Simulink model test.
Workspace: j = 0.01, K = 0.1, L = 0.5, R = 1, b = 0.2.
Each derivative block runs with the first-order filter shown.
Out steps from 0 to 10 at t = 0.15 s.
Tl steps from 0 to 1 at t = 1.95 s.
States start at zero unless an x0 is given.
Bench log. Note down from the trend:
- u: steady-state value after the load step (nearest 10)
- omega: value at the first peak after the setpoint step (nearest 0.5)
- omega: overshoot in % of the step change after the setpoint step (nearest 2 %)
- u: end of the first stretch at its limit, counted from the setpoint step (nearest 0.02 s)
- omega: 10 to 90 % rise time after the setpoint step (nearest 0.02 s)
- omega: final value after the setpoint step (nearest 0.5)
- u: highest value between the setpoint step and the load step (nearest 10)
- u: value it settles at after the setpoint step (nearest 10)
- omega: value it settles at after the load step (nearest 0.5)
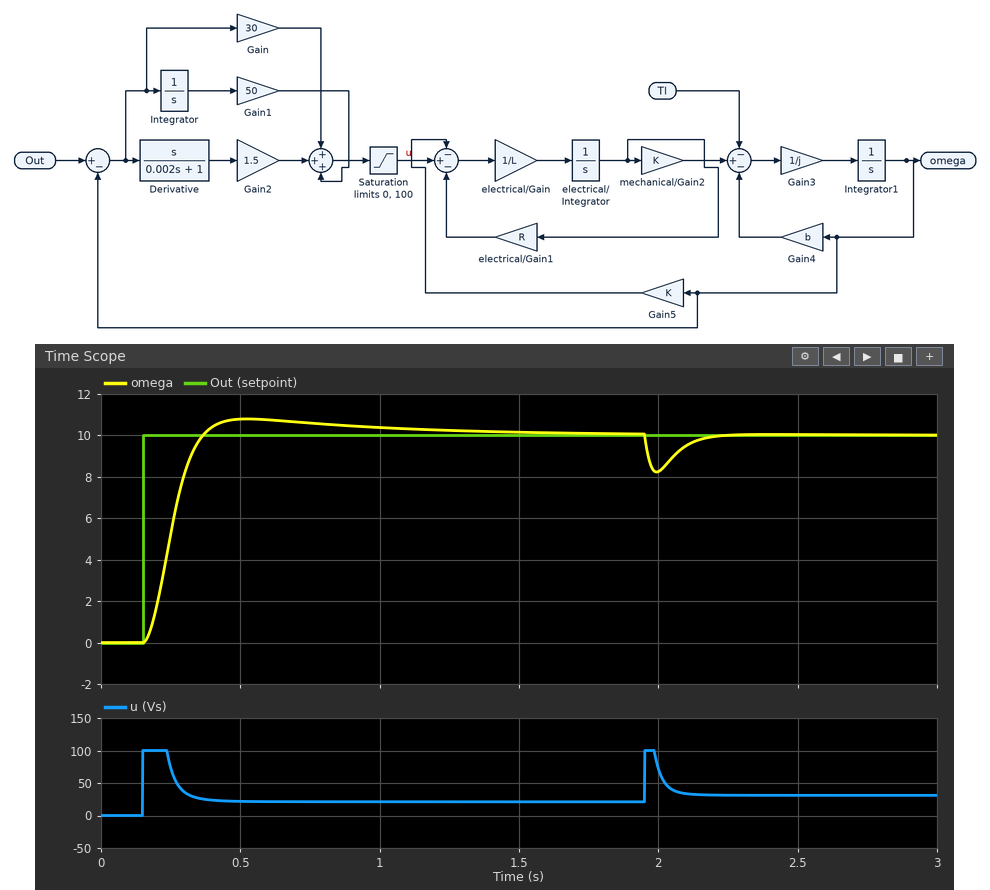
30
11.0
8 %
0.08 s
0.14 s
10.0
100
20
10.0
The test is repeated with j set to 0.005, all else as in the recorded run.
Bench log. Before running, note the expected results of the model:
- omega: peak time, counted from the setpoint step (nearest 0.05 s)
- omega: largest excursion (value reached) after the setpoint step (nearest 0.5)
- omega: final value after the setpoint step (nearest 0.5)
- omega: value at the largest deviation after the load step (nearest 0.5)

0.40 s
10.5
10.0
7.5
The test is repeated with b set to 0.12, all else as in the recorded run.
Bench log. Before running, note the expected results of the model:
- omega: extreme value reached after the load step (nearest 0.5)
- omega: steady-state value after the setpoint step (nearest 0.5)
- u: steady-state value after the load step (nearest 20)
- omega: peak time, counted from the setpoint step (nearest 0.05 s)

8.0
10.0
20
0.30 s
